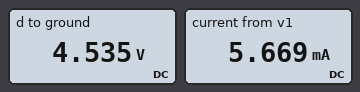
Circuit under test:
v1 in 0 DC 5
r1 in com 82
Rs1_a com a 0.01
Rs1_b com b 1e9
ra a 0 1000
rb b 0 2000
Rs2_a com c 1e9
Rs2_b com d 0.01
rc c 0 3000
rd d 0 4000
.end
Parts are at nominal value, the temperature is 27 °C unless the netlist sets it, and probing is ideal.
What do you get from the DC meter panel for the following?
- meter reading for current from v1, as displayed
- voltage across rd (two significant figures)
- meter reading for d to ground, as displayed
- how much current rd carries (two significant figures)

5.669 mA
4.5 V
4.535 V
1.1 mA
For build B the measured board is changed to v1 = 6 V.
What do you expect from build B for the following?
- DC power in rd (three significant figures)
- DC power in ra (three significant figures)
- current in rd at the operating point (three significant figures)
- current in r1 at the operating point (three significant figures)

7.40 mW
29.6 mW
1.36 mA
6.80 mA
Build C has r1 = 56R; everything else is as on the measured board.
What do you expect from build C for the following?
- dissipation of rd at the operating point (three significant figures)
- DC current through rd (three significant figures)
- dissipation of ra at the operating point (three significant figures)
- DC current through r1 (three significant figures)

5.46 mW
1.17 mA
21.8 mW
5.84 mA
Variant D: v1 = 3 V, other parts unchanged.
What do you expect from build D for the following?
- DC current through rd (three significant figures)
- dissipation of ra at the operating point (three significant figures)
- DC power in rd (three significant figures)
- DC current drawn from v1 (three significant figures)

680 µA
7.40 mW
1.85 mW
3.40 mA
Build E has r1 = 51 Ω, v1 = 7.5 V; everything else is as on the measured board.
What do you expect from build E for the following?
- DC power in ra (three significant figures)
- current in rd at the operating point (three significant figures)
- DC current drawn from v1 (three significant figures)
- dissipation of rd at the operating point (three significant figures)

49.7 mW
1.76 mA
8.81 mA
12.4 mW
